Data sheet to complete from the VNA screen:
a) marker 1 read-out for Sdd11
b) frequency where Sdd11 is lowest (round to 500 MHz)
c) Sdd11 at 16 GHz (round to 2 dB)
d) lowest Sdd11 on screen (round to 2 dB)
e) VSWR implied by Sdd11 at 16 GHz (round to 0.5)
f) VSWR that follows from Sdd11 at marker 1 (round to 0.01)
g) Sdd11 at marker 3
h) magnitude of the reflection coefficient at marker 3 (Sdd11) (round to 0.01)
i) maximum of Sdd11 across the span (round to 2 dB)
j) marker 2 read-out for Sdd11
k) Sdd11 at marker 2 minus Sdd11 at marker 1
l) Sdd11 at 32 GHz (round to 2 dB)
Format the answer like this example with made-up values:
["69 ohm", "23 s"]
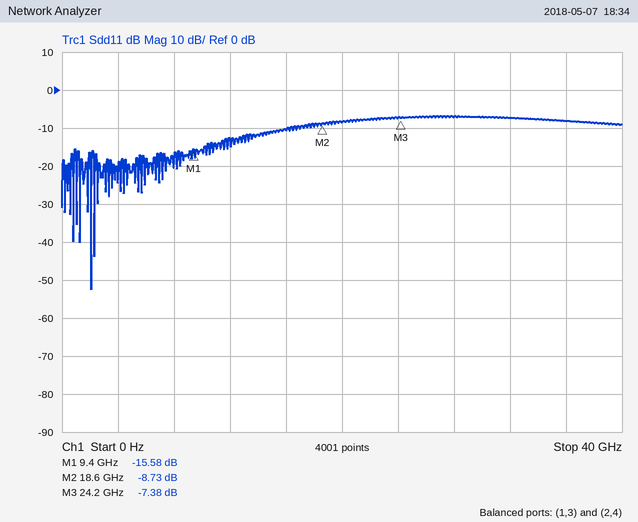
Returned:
["-15.58 dB", "2.0 GHz", "-10 dB", "-52 dB", "2.0", "1.40", "-7.38 dB", "0.43", "-6 dB", "-8.73 dB", "6.85 dB", "-8 dB"]
